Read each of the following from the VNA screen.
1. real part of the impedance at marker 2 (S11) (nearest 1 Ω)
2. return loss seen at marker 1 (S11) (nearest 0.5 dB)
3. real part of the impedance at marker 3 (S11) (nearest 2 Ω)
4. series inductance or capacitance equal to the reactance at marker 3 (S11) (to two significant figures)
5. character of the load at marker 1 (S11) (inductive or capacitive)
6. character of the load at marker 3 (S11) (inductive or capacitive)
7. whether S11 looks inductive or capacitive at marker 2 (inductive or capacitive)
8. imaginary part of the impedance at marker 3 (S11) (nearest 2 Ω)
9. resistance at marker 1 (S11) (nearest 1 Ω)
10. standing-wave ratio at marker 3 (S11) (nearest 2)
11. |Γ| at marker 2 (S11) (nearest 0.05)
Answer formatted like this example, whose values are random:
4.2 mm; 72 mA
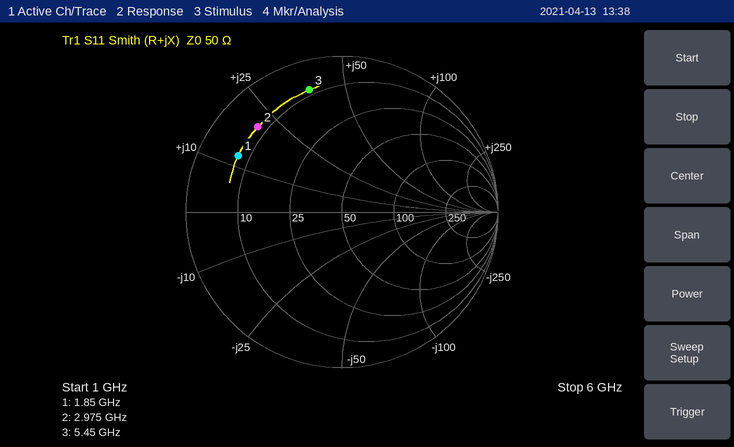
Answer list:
8 Ω; 2.5 dB; 8 Ω; 1.1 nH; inductive; inductive; inductive; +38 Ω; 7 Ω; 10; 0.75
